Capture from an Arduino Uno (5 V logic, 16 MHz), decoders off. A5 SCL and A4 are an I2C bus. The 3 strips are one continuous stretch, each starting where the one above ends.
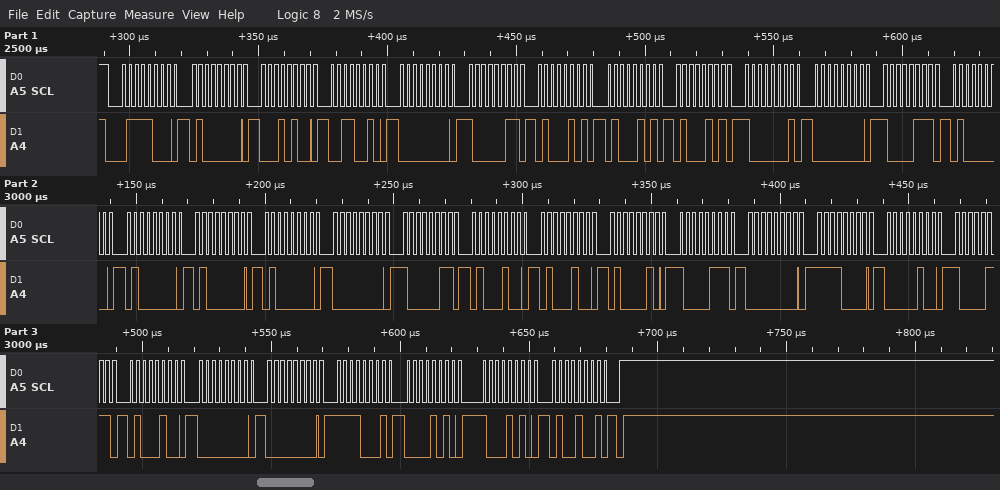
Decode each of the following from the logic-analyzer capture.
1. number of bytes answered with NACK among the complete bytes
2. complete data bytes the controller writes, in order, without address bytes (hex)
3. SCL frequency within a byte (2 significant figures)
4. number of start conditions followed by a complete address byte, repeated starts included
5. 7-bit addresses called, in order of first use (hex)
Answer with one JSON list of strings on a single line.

["0", "40 14 32 00 83 45 45 45 81 00 87 40 40 40 40 00 83 44 44 42 87 00 F0 04 87 44 00 00 F1 0A 8A 49", "400 kHz", "1", "0x3C"]
